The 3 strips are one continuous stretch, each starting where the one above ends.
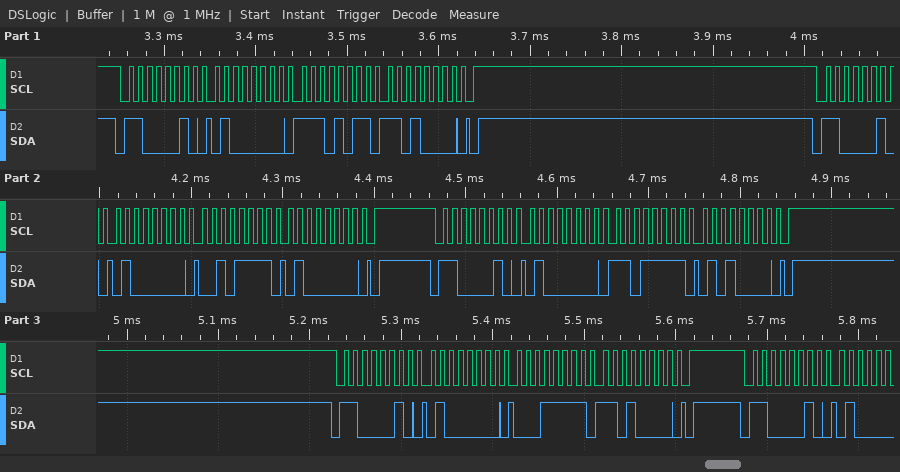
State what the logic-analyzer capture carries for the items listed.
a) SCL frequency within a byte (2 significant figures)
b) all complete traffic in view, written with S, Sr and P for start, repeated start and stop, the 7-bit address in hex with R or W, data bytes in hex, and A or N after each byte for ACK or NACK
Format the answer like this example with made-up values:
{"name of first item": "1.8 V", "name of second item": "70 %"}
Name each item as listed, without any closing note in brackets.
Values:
{"SCL frequency within a byte": "100 kHz", "all complete traffic in view, written with S, Sr and P for start, repeated start and stop, the 7-bit address in hex with R or W, data bytes in hex, and A or N after each byte for ACK or NACK": "S 61W A 40 A EB A D0 A P S 61W A 40 A 2F A 40 A P S 61W A 40 A DF A 50 A P S 61W A 40 A 1F A D0 A P S 61W A"}
